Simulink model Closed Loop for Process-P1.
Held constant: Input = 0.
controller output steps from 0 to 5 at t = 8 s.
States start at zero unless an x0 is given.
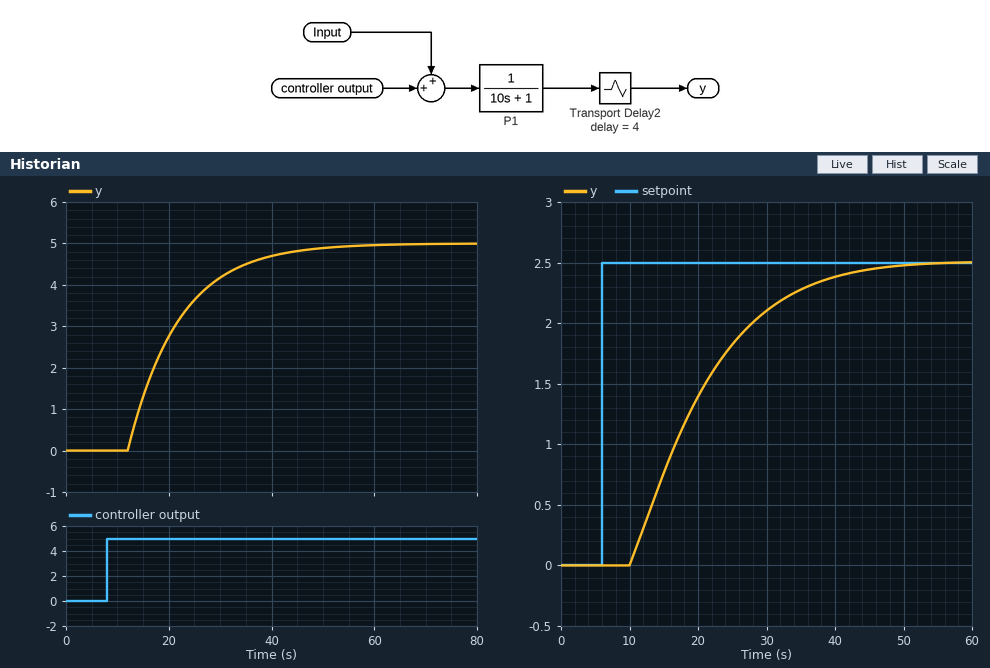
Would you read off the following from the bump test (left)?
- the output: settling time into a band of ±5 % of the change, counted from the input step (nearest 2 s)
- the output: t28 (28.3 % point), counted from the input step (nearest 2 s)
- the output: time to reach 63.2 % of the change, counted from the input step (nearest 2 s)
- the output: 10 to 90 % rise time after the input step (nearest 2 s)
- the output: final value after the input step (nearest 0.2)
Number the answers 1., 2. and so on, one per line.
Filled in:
1. 34 s
2. 8 s
3. 14 s
4. 22 s
5. 5.0
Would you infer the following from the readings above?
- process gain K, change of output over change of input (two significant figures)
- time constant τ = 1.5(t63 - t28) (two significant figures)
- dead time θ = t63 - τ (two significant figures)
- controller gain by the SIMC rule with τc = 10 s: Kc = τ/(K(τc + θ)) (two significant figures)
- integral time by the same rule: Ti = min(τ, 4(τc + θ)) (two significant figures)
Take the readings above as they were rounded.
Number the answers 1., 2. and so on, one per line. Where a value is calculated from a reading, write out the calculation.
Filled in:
1. (5 - 0) / 5 = 1.0
2. 1.5 × (14 - 8) = 9.0 s
3. 14 - 9 = 5.0 s
4. 9 / (1 × (10 + 5)) = 0.60
5. min(9, 4 × (10 + 5)) = 9.0 s
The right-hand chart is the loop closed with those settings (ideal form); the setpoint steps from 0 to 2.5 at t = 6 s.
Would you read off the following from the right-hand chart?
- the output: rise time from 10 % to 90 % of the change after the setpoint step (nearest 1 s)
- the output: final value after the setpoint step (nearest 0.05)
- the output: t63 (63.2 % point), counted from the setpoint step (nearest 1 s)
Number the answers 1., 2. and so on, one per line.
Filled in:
1. 22 s
2. 2.50
3. 16 s
